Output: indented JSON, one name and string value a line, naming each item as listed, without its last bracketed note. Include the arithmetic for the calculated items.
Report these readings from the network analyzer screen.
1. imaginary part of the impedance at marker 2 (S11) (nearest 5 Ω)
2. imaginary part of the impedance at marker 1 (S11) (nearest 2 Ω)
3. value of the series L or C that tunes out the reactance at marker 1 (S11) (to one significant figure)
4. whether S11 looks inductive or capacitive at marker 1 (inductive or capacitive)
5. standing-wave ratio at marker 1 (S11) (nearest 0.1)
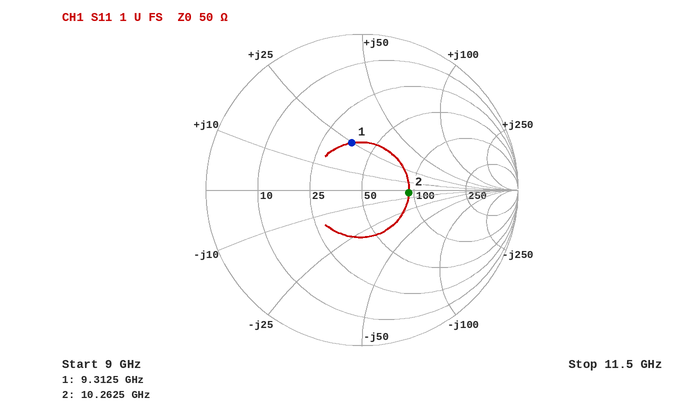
{
  "imaginary part of the impedance at marker 2 (S11)": "-5 Ω",
  "imaginary part of the impedance at marker 1 (S11)": "+24 Ω",
  "value of the series L or C that tunes out the reactance at marker 1 (S11)": "C = 1/(2π × 9.3125 GHz × 24 Ω) ≈ 712 fF, so 700 fF to one significant figure",
  "whether S11 looks inductive or capacitive at marker 1": "inductive",
  "standing-wave ratio at marker 1 (S11)": "1.9"
}
